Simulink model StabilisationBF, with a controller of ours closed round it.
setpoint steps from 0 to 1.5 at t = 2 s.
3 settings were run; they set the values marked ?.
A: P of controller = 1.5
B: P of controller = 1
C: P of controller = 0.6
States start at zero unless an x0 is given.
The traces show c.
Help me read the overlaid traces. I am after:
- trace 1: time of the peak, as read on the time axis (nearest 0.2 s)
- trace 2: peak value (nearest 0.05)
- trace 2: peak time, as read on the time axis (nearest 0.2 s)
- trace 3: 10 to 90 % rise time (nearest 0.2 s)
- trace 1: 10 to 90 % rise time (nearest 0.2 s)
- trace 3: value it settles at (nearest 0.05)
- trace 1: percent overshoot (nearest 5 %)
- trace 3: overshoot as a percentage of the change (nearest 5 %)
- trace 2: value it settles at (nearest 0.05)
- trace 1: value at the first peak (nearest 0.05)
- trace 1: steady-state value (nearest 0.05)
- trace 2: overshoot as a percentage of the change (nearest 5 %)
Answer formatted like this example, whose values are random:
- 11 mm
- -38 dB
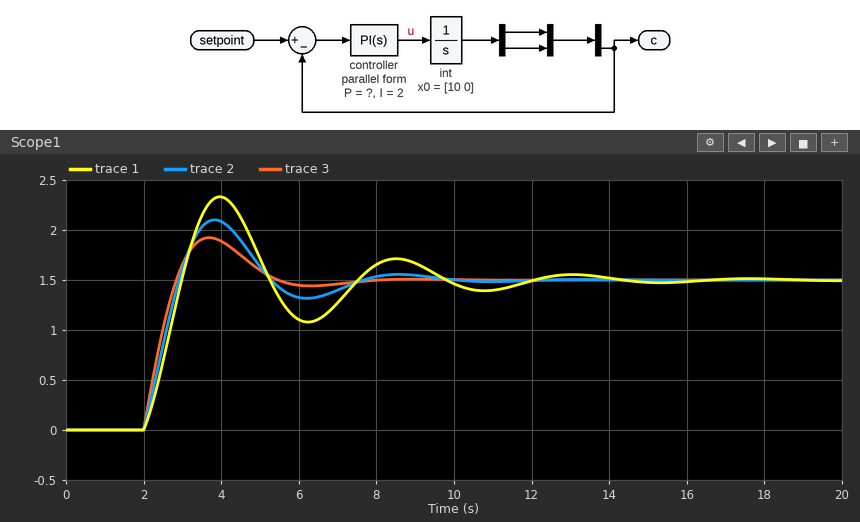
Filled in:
- 4.0 s
- 2.10
- 3.8 s
- 0.6 s
- 0.8 s
- 1.50
- 55 %
- 30 %
- 1.50
- 2.35
- 1.50
- 40 %
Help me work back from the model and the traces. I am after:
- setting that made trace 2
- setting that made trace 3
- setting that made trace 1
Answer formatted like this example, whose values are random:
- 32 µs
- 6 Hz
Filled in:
- B
- A
- C
